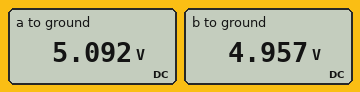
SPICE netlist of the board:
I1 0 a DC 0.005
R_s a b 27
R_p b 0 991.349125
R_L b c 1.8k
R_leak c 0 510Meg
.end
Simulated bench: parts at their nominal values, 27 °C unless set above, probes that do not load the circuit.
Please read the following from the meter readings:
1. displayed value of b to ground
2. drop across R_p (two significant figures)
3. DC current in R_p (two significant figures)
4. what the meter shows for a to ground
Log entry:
4.957 V
5.0 V
5.0 mA
5.092 V
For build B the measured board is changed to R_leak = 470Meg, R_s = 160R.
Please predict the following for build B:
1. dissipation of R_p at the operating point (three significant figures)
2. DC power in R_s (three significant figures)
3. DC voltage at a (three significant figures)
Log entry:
24.8 mW
4.00 mW
5.76 V
